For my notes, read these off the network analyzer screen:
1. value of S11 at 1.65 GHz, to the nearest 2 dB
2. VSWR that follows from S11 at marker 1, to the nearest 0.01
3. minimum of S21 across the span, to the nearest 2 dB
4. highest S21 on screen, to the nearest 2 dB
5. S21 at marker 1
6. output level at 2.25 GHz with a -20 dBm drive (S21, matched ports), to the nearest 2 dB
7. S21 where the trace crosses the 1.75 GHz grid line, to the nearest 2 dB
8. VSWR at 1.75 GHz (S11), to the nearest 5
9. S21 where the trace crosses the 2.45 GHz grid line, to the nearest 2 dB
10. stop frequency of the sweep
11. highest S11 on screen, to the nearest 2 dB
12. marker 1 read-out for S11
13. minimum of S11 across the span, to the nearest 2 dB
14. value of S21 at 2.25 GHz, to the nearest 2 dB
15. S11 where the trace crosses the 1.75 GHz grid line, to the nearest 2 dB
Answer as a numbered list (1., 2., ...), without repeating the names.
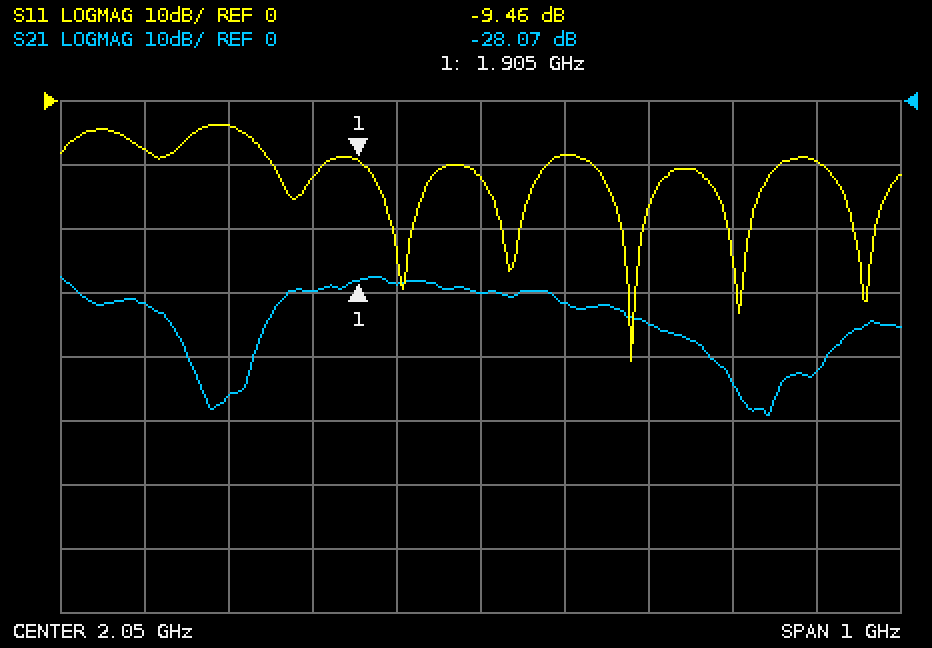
1. -8 dB
2. 2.01
3. -50 dB
4. -28 dB
5. -28.07 dB
6. -54 dBm
7. -46 dB
8. 5
9. -42 dB
10. 2.55 GHz
11. -4 dB
12. -9.46 dB
13. -40 dB
14. -34 dB
15. -4 dB
